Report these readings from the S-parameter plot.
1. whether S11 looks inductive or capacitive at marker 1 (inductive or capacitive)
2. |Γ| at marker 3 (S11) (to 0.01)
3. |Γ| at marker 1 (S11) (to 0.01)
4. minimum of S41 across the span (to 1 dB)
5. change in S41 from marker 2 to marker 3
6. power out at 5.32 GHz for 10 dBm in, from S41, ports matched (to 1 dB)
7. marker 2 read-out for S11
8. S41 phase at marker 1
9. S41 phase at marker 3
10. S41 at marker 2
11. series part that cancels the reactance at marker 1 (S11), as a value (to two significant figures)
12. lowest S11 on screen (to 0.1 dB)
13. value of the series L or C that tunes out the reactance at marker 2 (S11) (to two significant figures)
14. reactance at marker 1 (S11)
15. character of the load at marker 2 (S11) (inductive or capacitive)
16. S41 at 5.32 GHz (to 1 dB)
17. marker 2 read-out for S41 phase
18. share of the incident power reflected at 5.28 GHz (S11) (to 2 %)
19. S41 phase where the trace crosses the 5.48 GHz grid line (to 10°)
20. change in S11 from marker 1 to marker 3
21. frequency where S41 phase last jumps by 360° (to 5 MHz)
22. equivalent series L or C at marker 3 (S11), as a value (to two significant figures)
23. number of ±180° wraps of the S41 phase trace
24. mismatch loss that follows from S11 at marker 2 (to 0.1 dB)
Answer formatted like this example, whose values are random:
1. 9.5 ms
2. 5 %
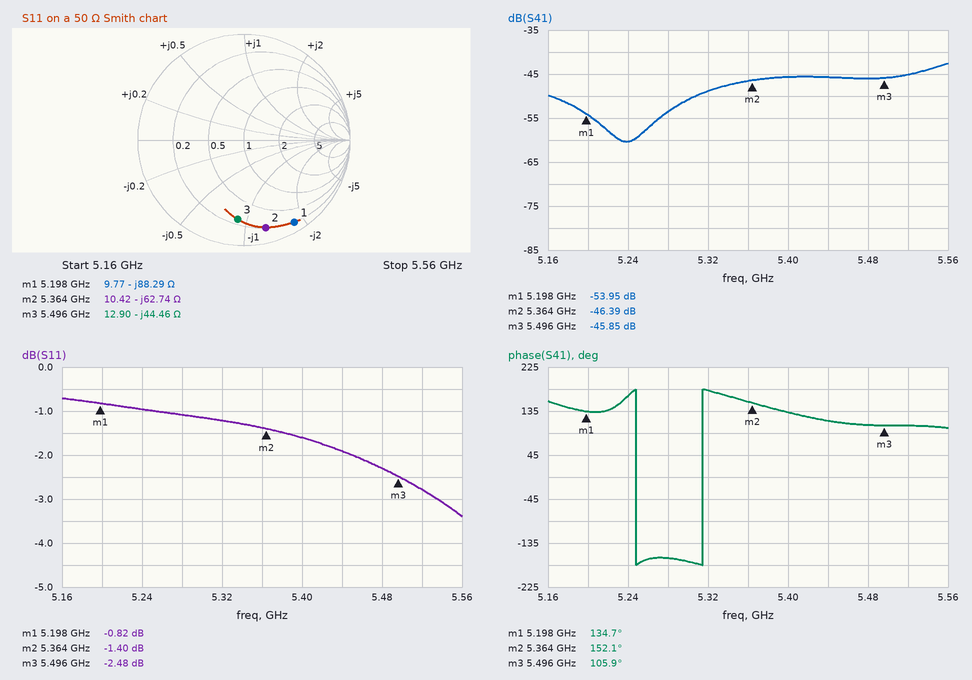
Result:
1. capacitive
2. 0.75
3. 0.91
4. -60 dB
5. 0.54 dB
6. -39 dBm
7. -1.40 dB
8. 134.7°
9. 105.9°
10. -46.39 dB
11. 2.7 nH
12. -3.4 dB
13. 1.9 nH
14. -88.29 Ω
15. capacitive
16. -49 dB
17. 152.1°
18. 78 %
19. 110°
20. -1.66 dB
21. 5.315 GHz
22. 650 fF
23. 2
24. 5.6 dB
